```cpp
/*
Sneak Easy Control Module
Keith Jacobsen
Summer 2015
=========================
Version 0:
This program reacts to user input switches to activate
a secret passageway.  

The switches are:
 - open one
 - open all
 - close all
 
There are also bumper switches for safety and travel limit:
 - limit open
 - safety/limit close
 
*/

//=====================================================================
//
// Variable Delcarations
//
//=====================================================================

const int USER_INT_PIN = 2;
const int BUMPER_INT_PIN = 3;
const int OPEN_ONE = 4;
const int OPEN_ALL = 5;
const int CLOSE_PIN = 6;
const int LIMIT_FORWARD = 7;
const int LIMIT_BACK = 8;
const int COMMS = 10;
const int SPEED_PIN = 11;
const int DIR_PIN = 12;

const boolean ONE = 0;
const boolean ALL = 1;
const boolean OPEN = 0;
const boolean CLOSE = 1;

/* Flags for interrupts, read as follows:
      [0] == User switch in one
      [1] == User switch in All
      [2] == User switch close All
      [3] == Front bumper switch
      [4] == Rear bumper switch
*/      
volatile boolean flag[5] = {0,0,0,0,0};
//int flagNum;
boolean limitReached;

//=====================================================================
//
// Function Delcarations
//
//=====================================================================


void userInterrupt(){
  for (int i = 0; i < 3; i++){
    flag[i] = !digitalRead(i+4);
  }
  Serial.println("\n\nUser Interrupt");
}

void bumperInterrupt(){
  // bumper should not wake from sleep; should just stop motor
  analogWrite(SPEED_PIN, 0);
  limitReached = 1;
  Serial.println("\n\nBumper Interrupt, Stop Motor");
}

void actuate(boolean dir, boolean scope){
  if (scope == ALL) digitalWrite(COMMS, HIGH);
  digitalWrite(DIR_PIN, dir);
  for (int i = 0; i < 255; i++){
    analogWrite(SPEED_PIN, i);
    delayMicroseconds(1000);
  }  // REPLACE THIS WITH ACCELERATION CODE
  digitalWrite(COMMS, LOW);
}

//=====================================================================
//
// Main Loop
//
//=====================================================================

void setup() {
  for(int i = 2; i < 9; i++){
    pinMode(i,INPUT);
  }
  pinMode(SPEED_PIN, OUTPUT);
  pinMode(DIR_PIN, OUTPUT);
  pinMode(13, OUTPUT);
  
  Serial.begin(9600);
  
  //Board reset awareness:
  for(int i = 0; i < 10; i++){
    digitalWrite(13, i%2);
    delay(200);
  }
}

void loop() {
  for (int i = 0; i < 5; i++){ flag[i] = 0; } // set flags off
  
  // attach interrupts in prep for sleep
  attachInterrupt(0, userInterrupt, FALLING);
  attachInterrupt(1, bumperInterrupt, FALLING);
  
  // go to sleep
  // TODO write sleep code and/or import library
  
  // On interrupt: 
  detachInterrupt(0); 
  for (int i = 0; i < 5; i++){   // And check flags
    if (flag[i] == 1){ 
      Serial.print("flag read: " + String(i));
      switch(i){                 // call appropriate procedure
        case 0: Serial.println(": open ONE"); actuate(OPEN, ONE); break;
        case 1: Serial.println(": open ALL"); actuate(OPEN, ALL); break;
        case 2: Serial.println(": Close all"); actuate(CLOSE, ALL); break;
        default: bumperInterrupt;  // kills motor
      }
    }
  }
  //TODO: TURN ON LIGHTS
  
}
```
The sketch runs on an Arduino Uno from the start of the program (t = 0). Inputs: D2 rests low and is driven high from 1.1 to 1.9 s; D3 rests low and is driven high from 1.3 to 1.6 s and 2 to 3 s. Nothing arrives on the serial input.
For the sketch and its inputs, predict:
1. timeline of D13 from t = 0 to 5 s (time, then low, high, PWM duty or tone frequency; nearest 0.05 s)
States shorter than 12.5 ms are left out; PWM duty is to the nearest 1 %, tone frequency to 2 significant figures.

0 s low; 0.2 s high; 0.4 s low; 0.6 s high; 0.8 s low; 1 s high; 1.2 s low; 1.4 s high; 1.6 s low; 1.8 s high
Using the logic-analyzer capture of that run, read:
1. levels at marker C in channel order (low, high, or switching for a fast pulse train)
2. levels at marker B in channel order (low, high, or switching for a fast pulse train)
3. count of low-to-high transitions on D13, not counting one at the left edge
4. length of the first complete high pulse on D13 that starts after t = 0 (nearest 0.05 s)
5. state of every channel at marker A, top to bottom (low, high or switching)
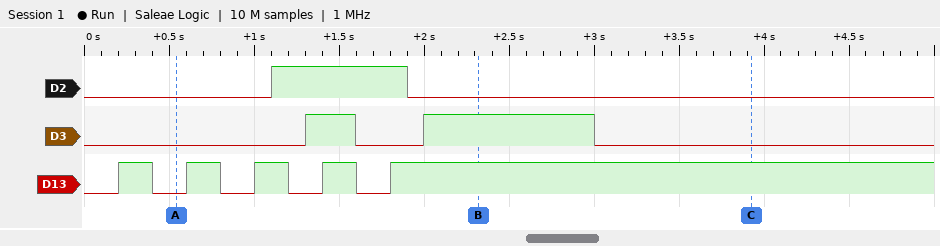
D2 low, D3 low, D13 high
D2 low, D3 high, D13 high
5
0.20 s
D2 low, D3 low, D13 low
